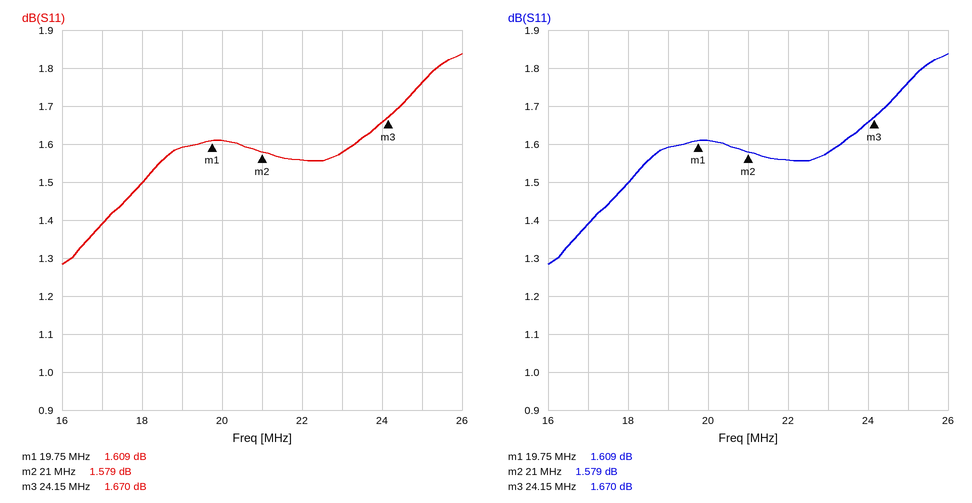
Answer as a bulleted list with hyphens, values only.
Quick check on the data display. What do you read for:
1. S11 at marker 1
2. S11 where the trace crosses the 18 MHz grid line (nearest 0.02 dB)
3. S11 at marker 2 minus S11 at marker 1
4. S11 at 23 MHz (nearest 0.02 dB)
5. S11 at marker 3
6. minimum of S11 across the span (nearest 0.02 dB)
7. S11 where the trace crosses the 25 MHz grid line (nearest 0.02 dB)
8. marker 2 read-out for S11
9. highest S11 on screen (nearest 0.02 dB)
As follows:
- 1.609 dB
- 1.50 dB
- -0.030 dB
- 1.58 dB
- 1.670 dB
- 1.28 dB
- 1.76 dB
- 1.579 dB
- 1.84 dB
